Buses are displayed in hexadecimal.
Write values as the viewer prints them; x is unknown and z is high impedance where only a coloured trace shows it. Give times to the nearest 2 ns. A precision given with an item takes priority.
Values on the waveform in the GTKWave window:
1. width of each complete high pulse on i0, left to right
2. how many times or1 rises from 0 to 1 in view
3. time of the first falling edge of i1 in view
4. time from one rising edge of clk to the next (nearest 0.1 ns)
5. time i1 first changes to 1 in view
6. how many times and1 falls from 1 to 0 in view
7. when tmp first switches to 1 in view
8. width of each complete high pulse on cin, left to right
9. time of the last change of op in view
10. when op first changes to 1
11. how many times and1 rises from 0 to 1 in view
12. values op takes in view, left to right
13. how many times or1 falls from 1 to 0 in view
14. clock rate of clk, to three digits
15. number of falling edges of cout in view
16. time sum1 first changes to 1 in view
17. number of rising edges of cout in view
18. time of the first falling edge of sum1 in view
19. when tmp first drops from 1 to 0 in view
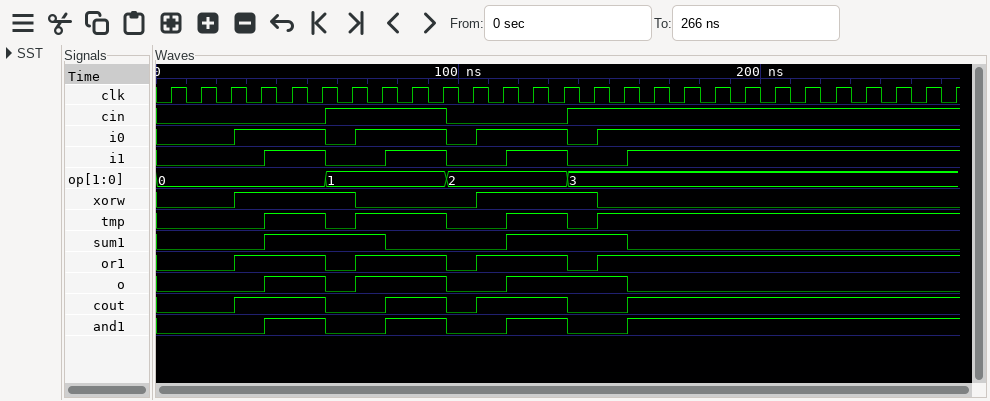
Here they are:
30 ns, 30 ns, 30 ns
4
56 ns
10 ns
36 ns
3
36 ns
40 ns
136 ns
56 ns
4
0, 1, 2, 3
3
100 MHz
3
36 ns
4
76 ns
56 ns
